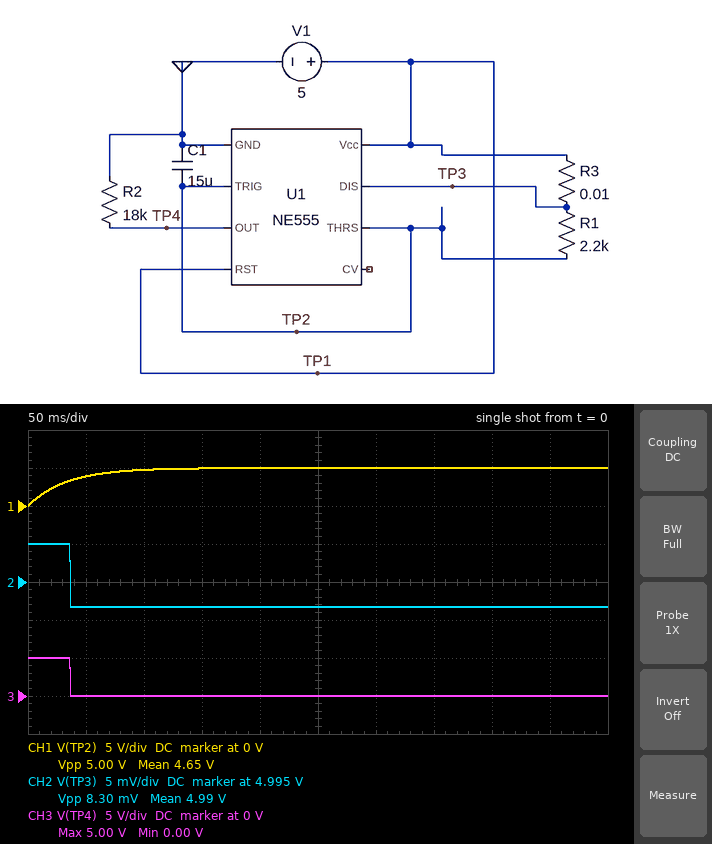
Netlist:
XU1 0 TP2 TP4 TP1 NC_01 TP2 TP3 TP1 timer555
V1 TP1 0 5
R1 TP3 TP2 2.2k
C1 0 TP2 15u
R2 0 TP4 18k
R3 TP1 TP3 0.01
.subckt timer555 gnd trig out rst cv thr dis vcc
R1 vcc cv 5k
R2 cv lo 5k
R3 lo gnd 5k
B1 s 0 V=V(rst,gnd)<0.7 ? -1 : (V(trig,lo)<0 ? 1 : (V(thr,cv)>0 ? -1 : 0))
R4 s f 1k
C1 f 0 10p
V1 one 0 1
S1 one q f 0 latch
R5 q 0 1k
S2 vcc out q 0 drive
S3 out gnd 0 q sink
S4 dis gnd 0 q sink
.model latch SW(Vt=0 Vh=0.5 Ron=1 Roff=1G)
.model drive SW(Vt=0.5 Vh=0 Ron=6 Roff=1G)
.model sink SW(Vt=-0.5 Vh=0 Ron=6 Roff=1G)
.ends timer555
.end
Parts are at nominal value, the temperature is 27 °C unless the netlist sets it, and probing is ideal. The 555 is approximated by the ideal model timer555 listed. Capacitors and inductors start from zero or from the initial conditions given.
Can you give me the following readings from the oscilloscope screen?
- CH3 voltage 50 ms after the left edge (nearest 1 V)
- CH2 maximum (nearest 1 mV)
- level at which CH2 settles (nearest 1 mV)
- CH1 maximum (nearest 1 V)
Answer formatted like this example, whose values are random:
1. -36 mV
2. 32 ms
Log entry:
1. 0 V
2. 5.000 V
3. 4.992 V
4. 5 V
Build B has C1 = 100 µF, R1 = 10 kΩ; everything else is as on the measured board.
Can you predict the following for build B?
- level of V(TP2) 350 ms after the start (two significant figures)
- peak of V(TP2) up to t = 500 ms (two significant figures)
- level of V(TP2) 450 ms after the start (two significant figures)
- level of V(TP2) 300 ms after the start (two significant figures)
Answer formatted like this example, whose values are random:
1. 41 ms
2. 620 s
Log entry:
1. 1.5 V
2. 2.0 V
3. 1.8 V
4. 1.3 V
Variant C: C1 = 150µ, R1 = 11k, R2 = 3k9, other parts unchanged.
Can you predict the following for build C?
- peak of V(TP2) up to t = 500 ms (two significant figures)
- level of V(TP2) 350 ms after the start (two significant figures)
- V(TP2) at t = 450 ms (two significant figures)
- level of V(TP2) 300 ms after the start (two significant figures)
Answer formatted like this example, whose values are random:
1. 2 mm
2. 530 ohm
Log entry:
1. 1.3 V
2. 960 mV
3. 1.2 V
4. 830 mV
